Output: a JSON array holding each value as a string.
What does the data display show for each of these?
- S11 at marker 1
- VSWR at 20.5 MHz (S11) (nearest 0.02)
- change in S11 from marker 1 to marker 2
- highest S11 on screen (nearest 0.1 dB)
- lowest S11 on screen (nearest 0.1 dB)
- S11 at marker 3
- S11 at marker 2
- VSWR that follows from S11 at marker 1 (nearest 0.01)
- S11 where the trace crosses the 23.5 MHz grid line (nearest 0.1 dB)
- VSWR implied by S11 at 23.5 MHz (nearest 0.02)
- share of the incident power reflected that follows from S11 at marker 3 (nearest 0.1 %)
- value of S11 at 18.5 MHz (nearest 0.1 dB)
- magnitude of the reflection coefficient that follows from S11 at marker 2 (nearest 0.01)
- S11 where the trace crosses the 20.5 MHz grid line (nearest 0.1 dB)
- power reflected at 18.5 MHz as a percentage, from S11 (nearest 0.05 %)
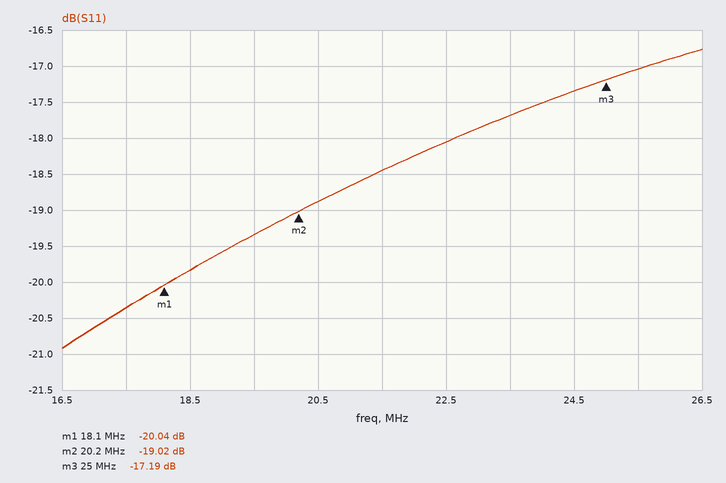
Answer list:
["-20.04 dB", "1.26", "1.02 dB", "-16.8 dB", "-20.9 dB", "-17.19 dB", "-19.02 dB", "1.22", "-17.7 dB", "1.30", "1.9 %", "-19.8 dB", "0.11", "-18.9 dB", "1.05 %"]
